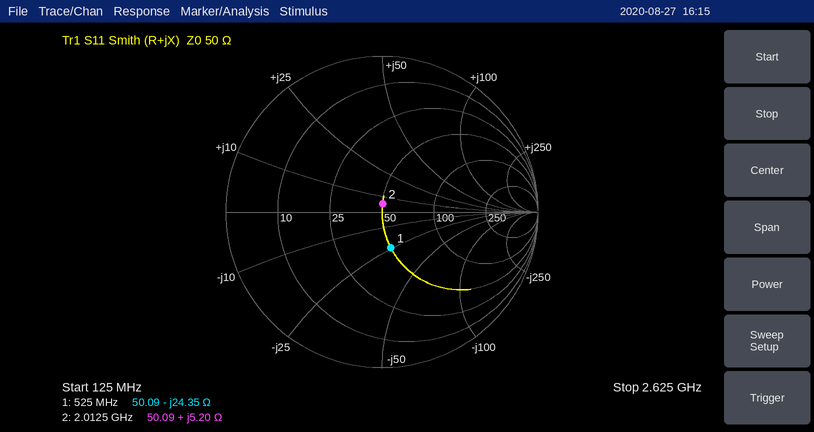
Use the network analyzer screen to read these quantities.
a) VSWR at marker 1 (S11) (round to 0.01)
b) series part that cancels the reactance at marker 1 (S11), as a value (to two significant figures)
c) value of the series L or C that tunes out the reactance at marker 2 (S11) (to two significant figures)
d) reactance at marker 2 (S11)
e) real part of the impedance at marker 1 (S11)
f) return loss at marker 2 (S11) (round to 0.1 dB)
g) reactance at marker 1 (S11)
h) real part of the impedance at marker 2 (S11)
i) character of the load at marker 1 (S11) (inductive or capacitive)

1.62
7.4 nH
15 pF
+5.20 Ω
50.09 Ω
25.7 dB
-24.35 Ω
50.09 Ω
capacitive
